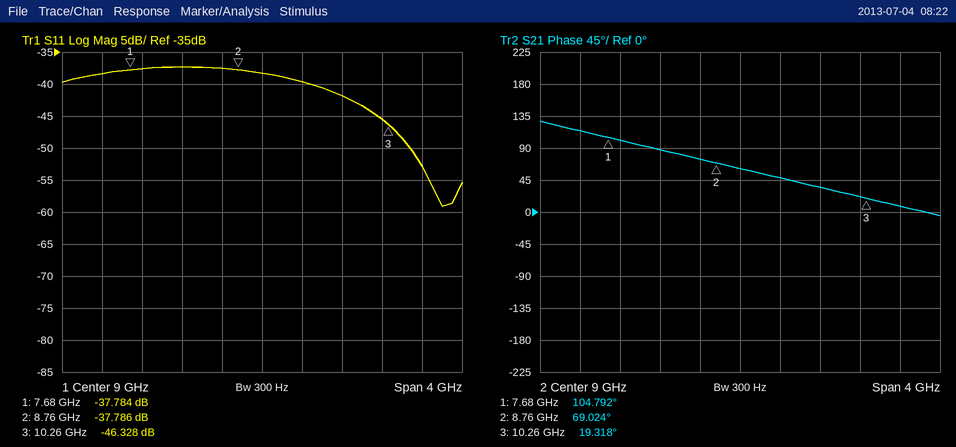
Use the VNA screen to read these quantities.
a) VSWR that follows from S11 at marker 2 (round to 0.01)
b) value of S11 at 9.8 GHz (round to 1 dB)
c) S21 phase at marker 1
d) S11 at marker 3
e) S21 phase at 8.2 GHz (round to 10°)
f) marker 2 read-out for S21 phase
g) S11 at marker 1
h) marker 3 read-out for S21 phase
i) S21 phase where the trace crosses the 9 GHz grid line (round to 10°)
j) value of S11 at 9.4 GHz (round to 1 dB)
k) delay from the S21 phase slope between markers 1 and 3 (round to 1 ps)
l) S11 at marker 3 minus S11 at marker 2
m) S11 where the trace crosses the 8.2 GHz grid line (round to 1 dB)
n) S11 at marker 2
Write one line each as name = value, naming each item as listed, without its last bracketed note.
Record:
VSWR that follows from S11 at marker 2 = 1.03
value of S11 at 9.8 GHz = -42 dB
S21 phase at marker 1 = 104.792°
S11 at marker 3 = -46.328 dB
S21 phase at 8.2 GHz = 90°
marker 2 read-out for S21 phase = 69.024°
S11 at marker 1 = -37.784 dB
marker 3 read-out for S21 phase = 19.318°
S21 phase where the trace crosses the 9 GHz grid line = 60°
value of S11 at 9.4 GHz = -40 dB
delay from the S21 phase slope between markers 1 and 3 = 92 ps
S11 at marker 3 minus S11 at marker 2 = -8.542 dB
S11 where the trace crosses the 8.2 GHz grid line = -37 dB
S11 at marker 2 = -37.786 dB
